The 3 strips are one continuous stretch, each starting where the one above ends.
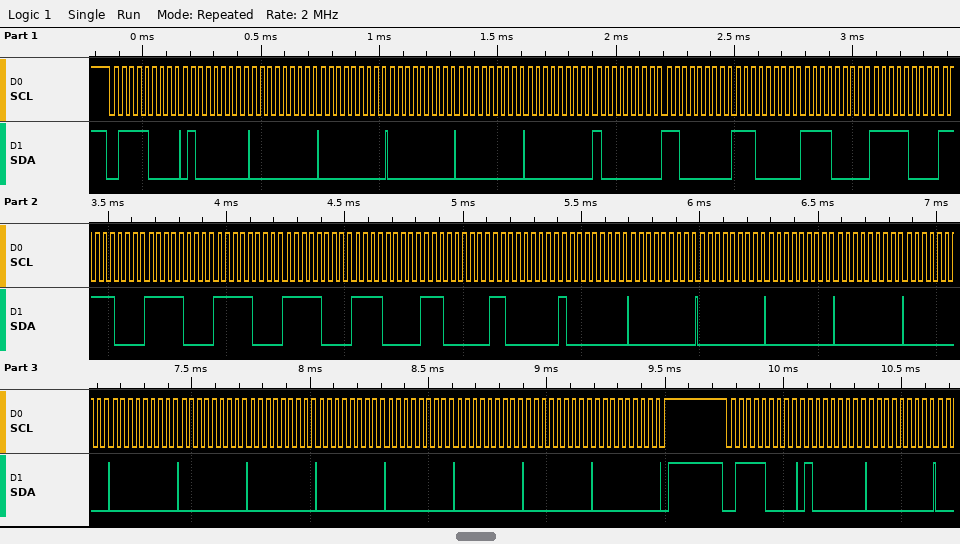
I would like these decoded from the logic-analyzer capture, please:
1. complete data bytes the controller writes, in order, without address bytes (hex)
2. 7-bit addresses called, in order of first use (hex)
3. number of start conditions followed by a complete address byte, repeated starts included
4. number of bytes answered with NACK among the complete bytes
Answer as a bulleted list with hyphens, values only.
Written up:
- 40 00 00 00 00 00 80 C0 E0 F0 F8 F8 F8 F8 F8 F0 E0 C0 80 00 00 00 00 00 00 00 00 00 00 00 00 00 40 00
- 0x3C
- 2
- 0
